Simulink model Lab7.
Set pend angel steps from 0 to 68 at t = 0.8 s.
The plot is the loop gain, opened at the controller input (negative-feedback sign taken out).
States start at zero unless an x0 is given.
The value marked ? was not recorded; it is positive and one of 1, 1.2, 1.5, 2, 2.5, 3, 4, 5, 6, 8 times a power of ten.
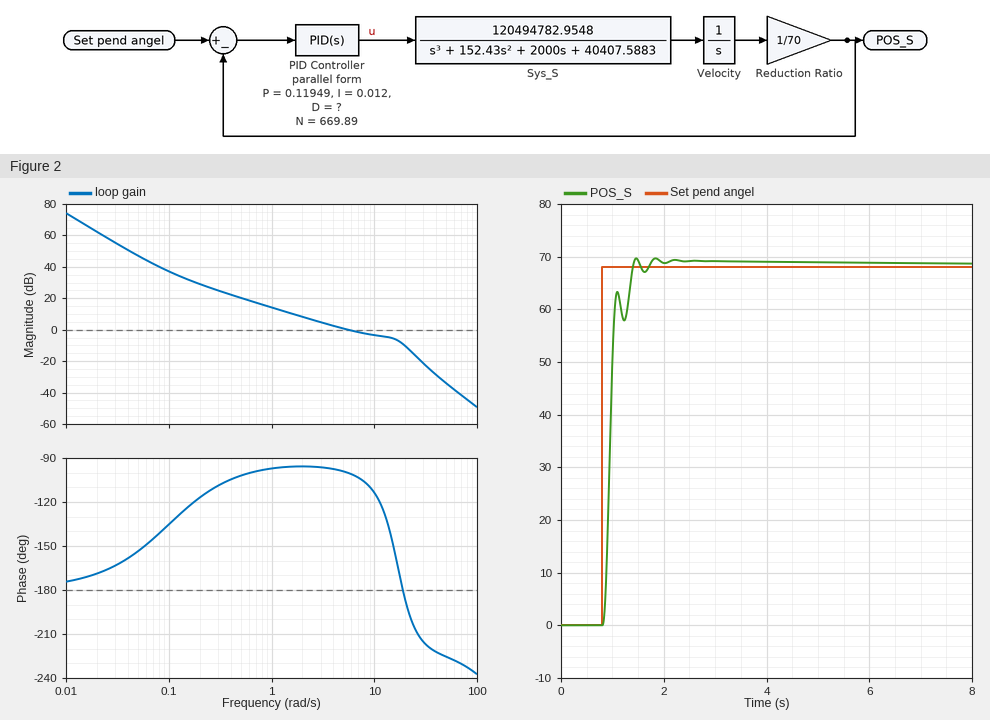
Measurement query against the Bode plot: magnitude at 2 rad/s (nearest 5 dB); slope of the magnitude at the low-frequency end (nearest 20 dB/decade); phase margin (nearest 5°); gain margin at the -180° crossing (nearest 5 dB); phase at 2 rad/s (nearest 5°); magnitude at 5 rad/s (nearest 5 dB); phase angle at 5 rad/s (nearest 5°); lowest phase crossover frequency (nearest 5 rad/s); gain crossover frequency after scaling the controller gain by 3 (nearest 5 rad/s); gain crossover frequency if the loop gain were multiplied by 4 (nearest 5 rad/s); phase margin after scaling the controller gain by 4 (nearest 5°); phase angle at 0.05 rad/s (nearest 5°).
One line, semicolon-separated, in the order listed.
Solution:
10 dB; -40 dB/decade; 80°; 10 dB; -95°; 0 dB; -100°; 20 rad/s; 20 rad/s; 20 rad/s; -15°; -155°
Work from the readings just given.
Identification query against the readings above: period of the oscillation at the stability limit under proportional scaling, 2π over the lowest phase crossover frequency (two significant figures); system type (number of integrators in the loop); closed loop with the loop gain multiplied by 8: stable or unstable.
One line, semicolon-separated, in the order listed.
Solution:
0.31 s; 2; unstable
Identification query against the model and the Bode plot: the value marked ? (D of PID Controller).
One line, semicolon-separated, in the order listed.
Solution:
0.003
